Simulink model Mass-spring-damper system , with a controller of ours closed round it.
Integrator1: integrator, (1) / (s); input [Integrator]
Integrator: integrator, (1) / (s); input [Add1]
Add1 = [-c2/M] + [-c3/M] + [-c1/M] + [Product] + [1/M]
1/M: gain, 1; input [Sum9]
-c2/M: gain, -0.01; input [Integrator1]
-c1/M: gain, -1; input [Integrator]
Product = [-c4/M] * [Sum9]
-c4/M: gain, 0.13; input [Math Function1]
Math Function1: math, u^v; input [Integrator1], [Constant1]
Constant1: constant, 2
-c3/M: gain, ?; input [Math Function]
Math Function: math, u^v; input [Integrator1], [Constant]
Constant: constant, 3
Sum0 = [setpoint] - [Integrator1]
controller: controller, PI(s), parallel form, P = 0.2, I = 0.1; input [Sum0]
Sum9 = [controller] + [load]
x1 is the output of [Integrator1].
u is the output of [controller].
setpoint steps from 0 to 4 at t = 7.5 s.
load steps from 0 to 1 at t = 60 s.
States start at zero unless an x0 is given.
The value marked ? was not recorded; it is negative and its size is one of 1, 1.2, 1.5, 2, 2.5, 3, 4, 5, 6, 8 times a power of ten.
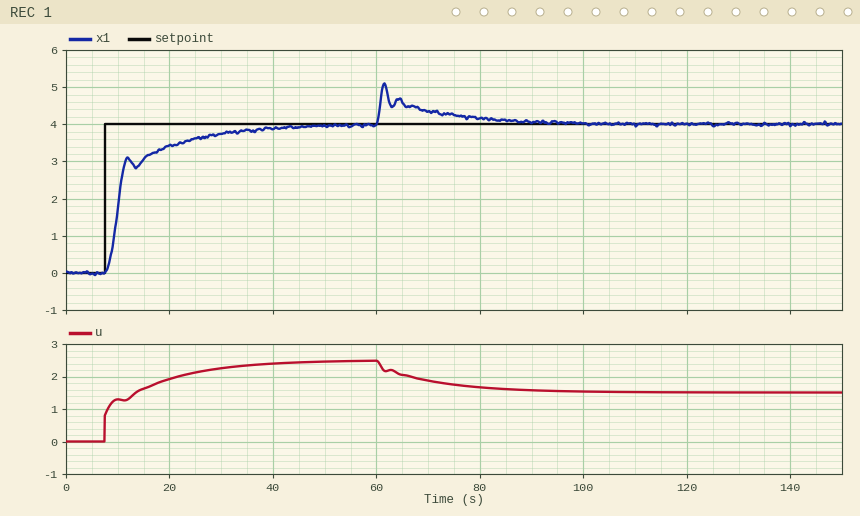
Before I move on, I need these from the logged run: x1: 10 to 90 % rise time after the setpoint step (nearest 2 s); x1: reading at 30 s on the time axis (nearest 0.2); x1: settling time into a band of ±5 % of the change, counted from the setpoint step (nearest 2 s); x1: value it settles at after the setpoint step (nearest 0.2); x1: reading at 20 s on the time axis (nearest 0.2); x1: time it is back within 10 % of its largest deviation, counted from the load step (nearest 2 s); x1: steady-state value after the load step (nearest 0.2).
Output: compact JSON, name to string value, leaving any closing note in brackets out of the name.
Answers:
{"x1: 10 to 90 % rise time after the setpoint step": "16 s", "x1: reading at 30 s on the time axis": "3.8", "x1: settling time into a band of ±5 % of the change, counted from the setpoint step": "26 s", "x1: value it settles at after the setpoint step": "4.0", "x1: reading at 20 s on the time axis": "3.4", "x1: time it is back within 10 % of its largest deviation, counted from the load step": "24 s", "x1: steady-state value after the load step": "4.0"}
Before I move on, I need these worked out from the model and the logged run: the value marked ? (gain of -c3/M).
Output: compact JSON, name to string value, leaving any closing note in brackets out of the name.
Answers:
{"the value marked ?": "-0.12"}
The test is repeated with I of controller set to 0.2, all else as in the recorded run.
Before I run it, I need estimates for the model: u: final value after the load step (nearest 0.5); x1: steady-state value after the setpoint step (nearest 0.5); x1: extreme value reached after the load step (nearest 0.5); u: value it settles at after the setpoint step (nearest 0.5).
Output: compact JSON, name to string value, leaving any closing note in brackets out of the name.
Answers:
{"u: final value after the load step": "1.5", "x1: steady-state value after the setpoint step": "4.0", "x1: extreme value reached after the load step": "5.0", "u: value it settles at after the setpoint step": "2.5"}
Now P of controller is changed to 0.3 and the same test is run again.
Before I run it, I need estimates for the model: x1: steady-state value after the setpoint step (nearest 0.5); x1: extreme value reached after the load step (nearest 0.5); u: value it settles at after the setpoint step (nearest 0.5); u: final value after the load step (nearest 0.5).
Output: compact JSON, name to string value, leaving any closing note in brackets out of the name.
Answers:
{"x1: steady-state value after the setpoint step": "4.0", "x1: extreme value reached after the load step": "5.0", "u: value it settles at after the setpoint step": "2.5", "u: final value after the load step": "1.5"}
